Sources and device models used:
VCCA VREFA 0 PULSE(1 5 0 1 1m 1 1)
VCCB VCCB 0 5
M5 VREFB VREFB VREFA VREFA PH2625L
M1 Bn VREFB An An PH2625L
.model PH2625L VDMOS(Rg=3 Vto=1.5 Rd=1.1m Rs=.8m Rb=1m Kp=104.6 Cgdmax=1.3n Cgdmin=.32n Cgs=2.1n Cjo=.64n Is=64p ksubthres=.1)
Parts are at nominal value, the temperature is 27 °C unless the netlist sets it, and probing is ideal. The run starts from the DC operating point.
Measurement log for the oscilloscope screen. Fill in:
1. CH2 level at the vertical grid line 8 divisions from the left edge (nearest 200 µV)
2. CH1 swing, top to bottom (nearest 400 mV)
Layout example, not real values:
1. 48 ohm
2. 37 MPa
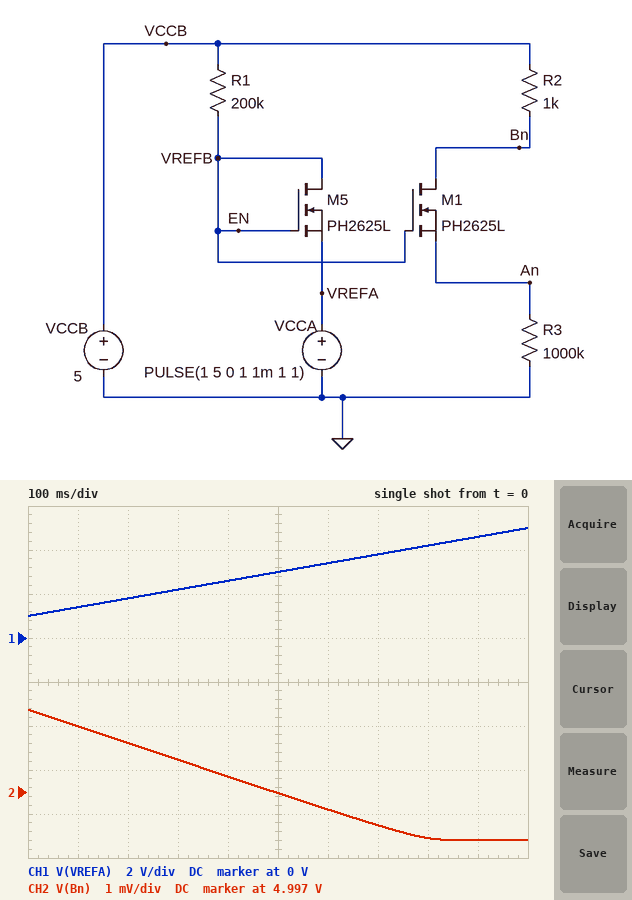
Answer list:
1. 4.9960 V
2. 4.0 V
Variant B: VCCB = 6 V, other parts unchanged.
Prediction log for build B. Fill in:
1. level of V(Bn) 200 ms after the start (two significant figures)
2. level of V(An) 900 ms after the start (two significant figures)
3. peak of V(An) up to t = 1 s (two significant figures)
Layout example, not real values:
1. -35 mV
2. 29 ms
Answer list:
1. 6.0 V
2. 4.6 V
3. 4.9 V
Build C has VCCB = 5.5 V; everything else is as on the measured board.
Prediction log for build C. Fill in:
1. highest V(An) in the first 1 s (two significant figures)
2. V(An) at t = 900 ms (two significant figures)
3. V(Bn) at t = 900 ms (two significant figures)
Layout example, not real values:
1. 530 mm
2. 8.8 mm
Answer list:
1. 4.6 V
2. 4.5 V
3. 5.5 V
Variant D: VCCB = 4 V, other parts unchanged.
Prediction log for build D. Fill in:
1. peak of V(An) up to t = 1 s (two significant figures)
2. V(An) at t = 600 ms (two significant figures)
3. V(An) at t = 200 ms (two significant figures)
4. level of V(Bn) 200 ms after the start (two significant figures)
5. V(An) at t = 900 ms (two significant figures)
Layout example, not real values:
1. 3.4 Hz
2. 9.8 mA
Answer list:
1. 3.8 V
2. 3.1 V
3. 1.9 V
4. 4.0 V
5. 3.4 V
